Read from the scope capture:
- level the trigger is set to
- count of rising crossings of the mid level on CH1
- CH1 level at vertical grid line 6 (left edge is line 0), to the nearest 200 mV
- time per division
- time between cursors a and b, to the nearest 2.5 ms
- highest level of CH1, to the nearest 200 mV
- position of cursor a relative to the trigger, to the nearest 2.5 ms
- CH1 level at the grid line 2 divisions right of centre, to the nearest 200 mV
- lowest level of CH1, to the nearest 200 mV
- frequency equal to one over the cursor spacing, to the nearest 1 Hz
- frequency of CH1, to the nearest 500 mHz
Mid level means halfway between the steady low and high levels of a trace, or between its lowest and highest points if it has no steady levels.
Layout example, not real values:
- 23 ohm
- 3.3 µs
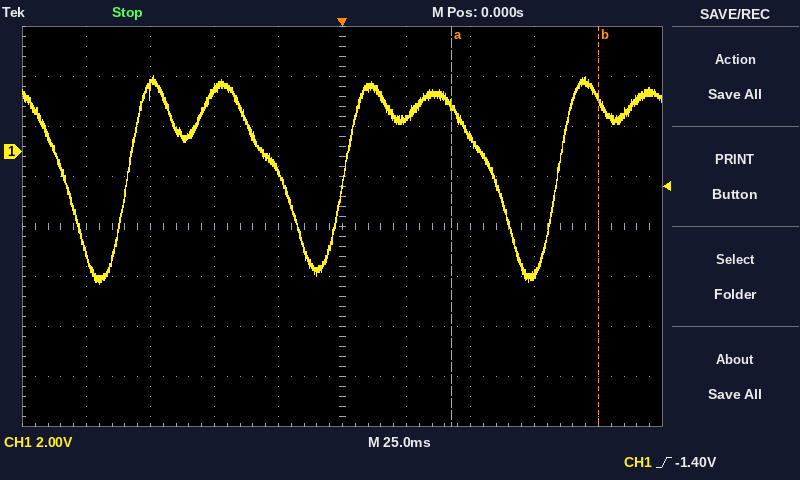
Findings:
- -1.40 V
- 3
- 1.2 V
- 25 ms
- 57.5 ms
- 3.0 V
- +42.5 ms
- 600 mV
- -5.2 V
- 17 Hz
- 12.0 Hz
